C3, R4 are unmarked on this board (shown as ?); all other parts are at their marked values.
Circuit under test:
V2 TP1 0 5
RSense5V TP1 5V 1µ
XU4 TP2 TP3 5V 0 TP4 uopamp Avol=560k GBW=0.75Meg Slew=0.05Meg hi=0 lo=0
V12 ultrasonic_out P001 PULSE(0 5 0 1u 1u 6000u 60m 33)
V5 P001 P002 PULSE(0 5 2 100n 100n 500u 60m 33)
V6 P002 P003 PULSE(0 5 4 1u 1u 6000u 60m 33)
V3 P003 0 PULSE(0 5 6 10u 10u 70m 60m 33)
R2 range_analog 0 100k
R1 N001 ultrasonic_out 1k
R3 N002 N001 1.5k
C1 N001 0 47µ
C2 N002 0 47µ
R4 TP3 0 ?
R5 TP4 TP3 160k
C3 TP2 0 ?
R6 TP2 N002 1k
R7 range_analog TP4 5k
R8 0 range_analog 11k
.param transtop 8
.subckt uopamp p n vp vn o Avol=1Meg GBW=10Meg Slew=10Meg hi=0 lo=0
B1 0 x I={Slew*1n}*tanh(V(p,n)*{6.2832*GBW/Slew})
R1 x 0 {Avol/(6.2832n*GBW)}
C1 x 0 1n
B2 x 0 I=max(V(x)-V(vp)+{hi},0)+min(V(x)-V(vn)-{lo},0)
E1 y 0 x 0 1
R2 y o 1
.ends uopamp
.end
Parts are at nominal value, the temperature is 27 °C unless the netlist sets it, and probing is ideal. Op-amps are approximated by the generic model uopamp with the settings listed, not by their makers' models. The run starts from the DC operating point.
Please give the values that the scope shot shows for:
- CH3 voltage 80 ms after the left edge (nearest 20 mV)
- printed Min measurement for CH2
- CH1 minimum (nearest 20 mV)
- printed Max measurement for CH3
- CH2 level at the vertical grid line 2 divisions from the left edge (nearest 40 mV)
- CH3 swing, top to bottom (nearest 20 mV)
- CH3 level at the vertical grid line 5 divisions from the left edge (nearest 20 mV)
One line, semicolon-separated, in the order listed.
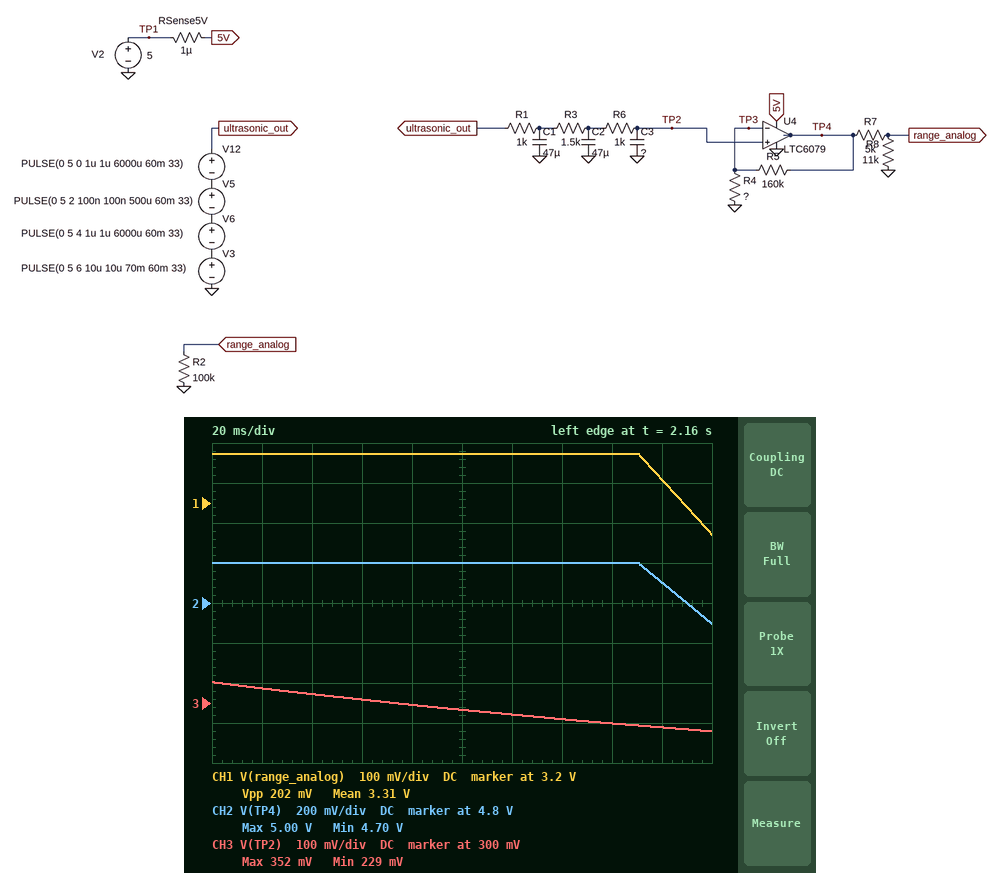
300 mV; 4.70 V; 3.12 V; 352 mV; 5.00 V; 120 mV; 280 mV
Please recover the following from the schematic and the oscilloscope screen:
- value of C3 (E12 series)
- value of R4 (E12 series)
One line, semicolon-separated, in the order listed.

82 µF; 8.2 kΩ
